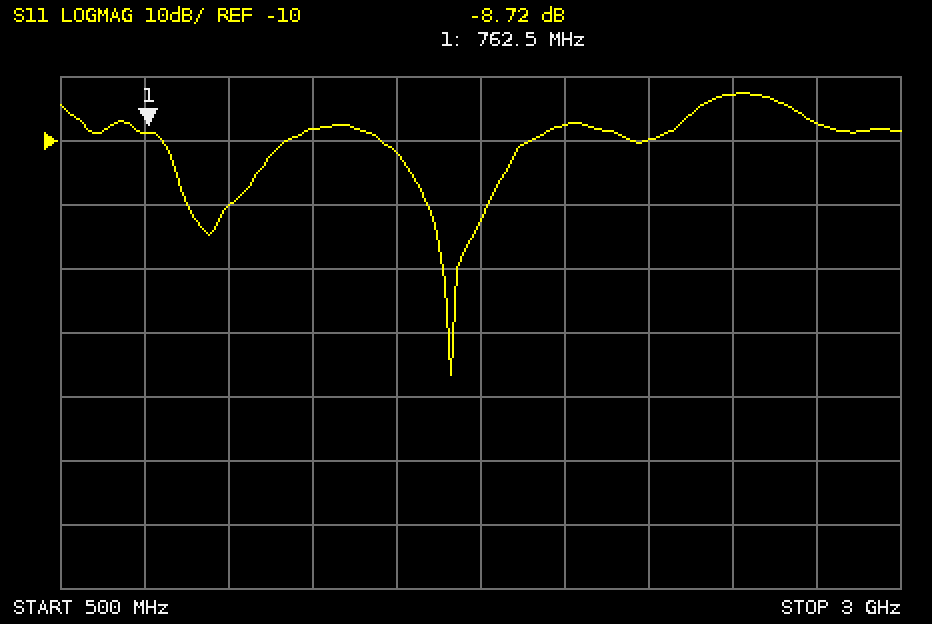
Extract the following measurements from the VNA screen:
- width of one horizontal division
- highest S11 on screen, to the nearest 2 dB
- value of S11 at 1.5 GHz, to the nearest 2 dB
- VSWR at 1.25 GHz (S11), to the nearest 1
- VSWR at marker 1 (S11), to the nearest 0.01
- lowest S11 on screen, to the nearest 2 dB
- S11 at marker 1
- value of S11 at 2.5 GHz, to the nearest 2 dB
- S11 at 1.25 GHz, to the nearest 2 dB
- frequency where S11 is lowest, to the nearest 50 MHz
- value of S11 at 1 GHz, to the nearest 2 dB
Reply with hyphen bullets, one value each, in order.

- 250 MHz
- -2 dB
- -12 dB
- 2
- 2.16
- -46 dB
- -8.72 dB
- -2 dB
- -8 dB
- 1.65 GHz
- -20 dB
